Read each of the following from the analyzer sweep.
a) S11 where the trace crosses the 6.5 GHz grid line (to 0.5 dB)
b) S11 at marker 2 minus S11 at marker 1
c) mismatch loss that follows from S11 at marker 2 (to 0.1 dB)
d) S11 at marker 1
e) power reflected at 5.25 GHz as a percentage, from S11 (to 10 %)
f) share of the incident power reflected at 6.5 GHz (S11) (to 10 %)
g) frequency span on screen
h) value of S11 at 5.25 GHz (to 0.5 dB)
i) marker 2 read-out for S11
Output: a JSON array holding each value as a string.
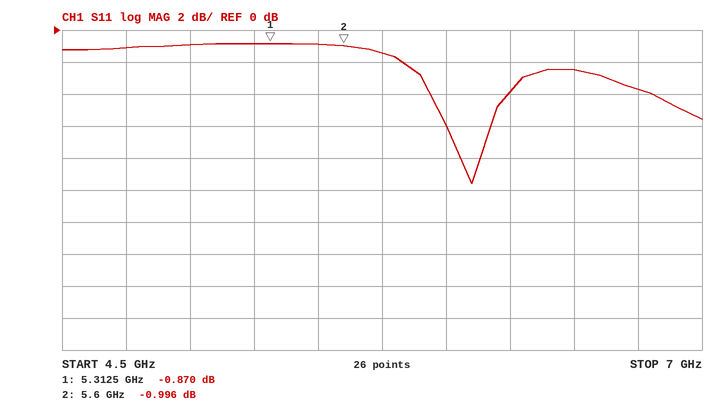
["-2.5 dB", "-0.126 dB", "6.9 dB", "-0.870 dB", "80 %", "60 %", "2.5 GHz", "-1.0 dB", "-0.996 dB"]
